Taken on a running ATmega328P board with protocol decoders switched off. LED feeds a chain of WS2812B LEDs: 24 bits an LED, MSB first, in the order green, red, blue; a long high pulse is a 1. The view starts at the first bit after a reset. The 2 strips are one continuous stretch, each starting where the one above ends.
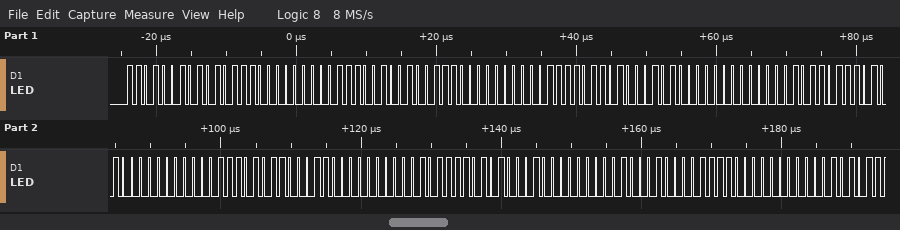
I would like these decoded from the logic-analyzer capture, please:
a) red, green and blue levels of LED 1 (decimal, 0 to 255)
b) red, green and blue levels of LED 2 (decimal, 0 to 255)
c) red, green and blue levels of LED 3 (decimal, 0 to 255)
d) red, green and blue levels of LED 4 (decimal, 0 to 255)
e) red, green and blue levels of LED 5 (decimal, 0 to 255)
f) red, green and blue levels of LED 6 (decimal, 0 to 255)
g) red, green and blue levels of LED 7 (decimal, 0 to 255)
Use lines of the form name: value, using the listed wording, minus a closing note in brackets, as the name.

red, green and blue levels of LED 1: 174, 210, 0
red, green and blue levels of LED 2: 156, 228, 0
red, green and blue levels of LED 3: 138, 246, 0
red, green and blue levels of LED 4: 117, 11, 0
red, green and blue levels of LED 5: 99, 29, 0
red, green and blue levels of LED 6: 81, 47, 0
red, green and blue levels of LED 7: 60, 68, 0
